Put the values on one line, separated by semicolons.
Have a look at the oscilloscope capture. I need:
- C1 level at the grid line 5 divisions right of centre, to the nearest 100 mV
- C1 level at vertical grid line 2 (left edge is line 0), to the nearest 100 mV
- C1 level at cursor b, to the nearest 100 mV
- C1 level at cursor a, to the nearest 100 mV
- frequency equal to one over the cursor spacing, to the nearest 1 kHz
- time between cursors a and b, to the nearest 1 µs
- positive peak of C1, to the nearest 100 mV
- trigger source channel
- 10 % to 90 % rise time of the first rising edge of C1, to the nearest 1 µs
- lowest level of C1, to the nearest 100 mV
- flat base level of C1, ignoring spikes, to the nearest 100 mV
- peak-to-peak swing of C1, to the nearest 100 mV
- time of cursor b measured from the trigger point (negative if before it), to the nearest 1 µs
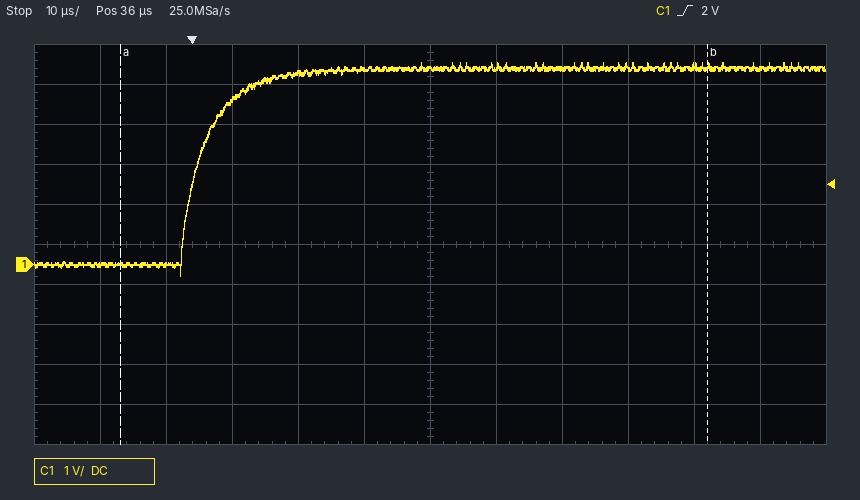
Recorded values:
4.9 V; 0.0 V; 4.9 V; 0.0 V; 11 kHz; 89 µs; 5.0 V; C1; 10 µs; -300 mV; 0.0 V; 5.3 V; +78 µs
